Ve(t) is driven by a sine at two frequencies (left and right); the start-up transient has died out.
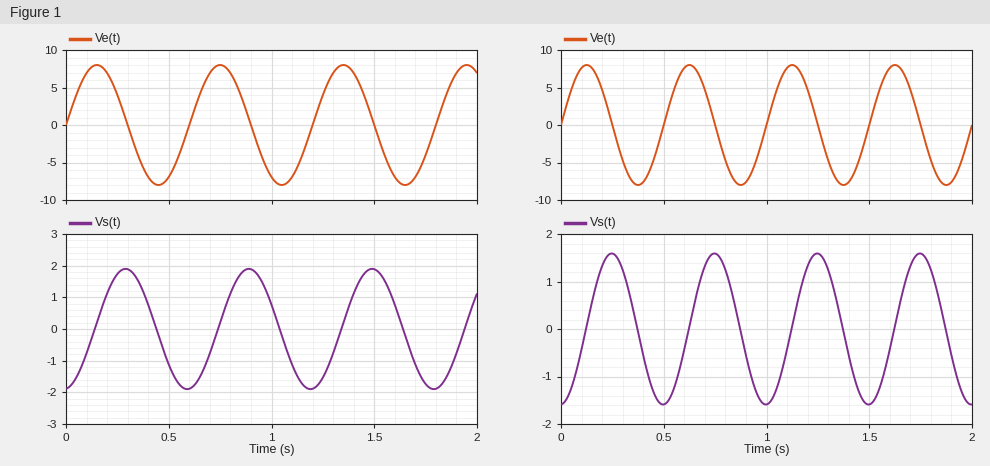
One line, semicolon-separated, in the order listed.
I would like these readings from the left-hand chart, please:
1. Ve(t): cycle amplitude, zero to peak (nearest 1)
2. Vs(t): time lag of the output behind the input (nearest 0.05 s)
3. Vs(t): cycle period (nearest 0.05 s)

8; 0.15 s; 0.60 s
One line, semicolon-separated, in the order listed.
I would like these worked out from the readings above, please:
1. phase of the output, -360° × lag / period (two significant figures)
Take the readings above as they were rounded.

-90°
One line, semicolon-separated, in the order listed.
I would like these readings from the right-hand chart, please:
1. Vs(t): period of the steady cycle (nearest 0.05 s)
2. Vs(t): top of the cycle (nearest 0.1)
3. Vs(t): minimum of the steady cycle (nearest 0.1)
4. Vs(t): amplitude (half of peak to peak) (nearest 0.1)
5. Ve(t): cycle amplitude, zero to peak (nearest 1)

0.50 s; 1.6; -1.6; 1.6; 8
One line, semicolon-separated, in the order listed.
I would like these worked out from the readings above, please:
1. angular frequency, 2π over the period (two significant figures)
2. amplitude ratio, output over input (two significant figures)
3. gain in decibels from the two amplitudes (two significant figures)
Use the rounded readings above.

13 rad/s; 0.20; -14 dB
